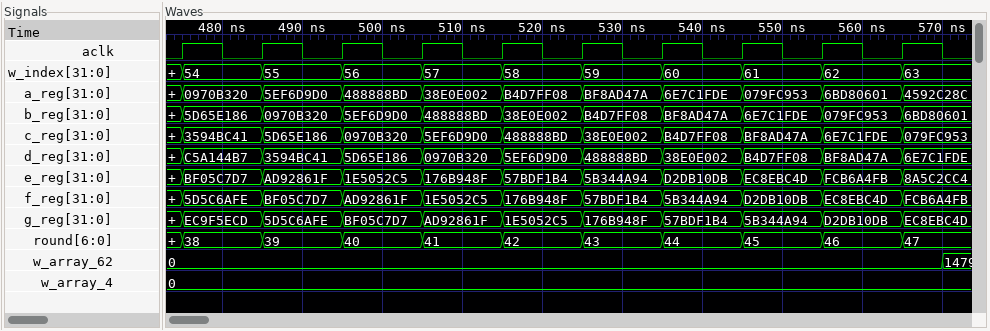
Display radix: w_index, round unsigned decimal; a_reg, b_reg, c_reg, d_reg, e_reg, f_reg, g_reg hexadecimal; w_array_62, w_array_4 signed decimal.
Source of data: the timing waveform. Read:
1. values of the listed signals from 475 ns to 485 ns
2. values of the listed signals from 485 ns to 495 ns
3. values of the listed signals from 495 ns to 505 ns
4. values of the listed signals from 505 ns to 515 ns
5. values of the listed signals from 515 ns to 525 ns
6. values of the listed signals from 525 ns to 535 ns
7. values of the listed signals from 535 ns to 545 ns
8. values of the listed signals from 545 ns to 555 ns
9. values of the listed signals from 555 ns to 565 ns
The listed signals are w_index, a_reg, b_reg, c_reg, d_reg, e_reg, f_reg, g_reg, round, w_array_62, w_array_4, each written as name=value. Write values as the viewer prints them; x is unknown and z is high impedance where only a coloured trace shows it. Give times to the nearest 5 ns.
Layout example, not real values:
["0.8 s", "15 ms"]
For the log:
["w_index=54, a_reg=0970B320, b_reg=5D65E186, c_reg=3594BC41, d_reg=C5A144B7, e_reg=BF05C7D7, f_reg=5D5C6AFE, g_reg=EC9F5ECD, round=38, w_array_62=0, w_array_4=0", "w_index=55, a_reg=5EF6D9D0, b_reg=0970B320, c_reg=5D65E186, d_reg=3594BC41, e_reg=AD92861F, f_reg=BF05C7D7, g_reg=5D5C6AFE, round=39, w_array_62=0, w_array_4=0", "w_index=56, a_reg=488888BD, b_reg=5EF6D9D0, c_reg=0970B320, d_reg=5D65E186, e_reg=1E5052C5, f_reg=AD92861F, g_reg=BF05C7D7, round=40, w_array_62=0, w_array_4=0", "w_index=57, a_reg=38E0E002, b_reg=488888BD, c_reg=5EF6D9D0, d_reg=0970B320, e_reg=176B948F, f_reg=1E5052C5, g_reg=AD92861F, round=41, w_array_62=0, w_array_4=0", "w_index=58, a_reg=B4D7FF08, b_reg=38E0E002, c_reg=488888BD, d_reg=5EF6D9D0, e_reg=57BDF1B4, f_reg=176B948F, g_reg=1E5052C5, round=42, w_array_62=0, w_array_4=0", "w_index=59, a_reg=BF8AD47A, b_reg=B4D7FF08, c_reg=38E0E002, d_reg=488888BD, e_reg=5B344A94, f_reg=57BDF1B4, g_reg=176B948F, round=43, w_array_62=0, w_array_4=0", "w_index=60, a_reg=6E7C1FDE, b_reg=BF8AD47A, c_reg=B4D7FF08, d_reg=38E0E002, e_reg=D2DB10DB, f_reg=5B344A94, g_reg=57BDF1B4, round=44, w_array_62=0, w_array_4=0", "w_index=61, a_reg=079FC953, b_reg=6E7C1FDE, c_reg=BF8AD47A, d_reg=B4D7FF08, e_reg=EC8EBC4D, f_reg=D2DB10DB, g_reg=5B344A94, round=45, w_array_62=0, w_array_4=0", "w_index=62, a_reg=6BD80601, b_reg=079FC953, c_reg=6E7C1FDE, d_reg=BF8AD47A, e_reg=FCB6A4FB, f_reg=EC8EBC4D, g_reg=D2DB10DB, round=46, w_array_62=0, w_array_4=0"]
